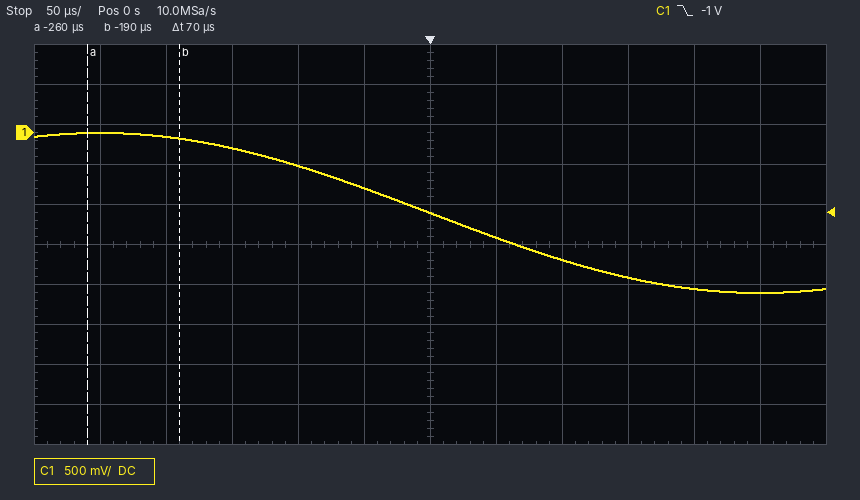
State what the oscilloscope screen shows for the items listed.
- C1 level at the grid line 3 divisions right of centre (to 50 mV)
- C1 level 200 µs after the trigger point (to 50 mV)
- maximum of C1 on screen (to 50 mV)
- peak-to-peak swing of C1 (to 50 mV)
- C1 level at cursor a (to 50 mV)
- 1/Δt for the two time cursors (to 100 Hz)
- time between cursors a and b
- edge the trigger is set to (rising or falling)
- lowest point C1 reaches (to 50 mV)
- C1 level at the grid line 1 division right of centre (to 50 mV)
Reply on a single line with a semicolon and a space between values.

-1.80 V; -1.95 V; 0 mV; 2.00 V; 0 mV; 14.3 kHz; 70 µs; falling; -2.00 V; -1.30 V
